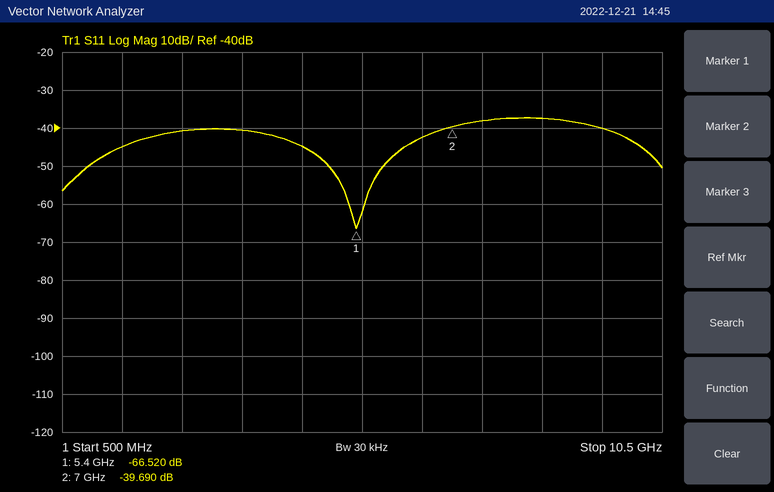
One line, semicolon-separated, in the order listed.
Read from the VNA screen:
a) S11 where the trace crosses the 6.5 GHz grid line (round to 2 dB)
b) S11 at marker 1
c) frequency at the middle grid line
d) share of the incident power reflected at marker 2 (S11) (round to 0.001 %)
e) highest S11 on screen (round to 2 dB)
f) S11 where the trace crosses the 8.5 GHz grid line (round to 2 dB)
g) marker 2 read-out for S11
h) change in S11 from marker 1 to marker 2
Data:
-42 dB; -66.520 dB; 5.5 GHz; 0.011 %; -38 dB; -38 dB; -39.690 dB; 26.830 dB
